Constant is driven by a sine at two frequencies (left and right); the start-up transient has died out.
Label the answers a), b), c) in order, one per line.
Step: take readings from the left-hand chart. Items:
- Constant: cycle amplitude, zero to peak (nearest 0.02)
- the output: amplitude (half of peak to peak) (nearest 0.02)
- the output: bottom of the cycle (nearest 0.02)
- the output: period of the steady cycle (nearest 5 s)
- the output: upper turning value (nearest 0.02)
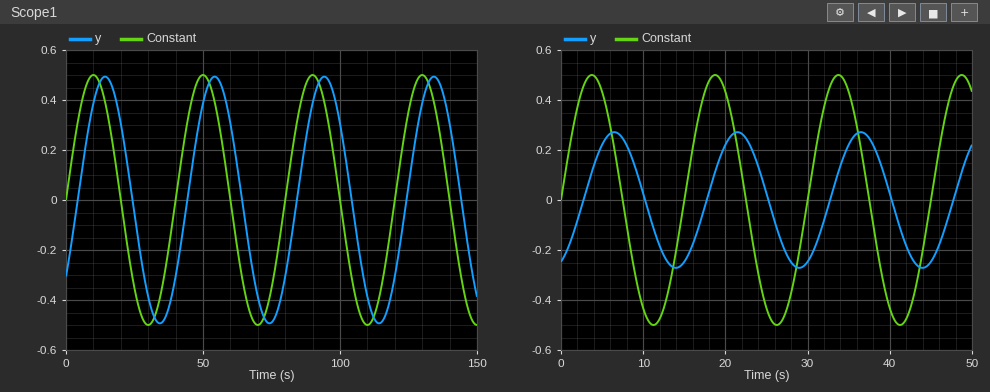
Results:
a) 0.50
b) 0.50
c) -0.50
d) 40 s
e) 0.50
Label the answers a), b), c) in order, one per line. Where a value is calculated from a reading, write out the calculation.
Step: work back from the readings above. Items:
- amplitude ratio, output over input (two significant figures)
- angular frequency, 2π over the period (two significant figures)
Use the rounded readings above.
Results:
a) 0.5 / 0.5 = 1.0
b) 2π / 40 = 0.16 rad/s
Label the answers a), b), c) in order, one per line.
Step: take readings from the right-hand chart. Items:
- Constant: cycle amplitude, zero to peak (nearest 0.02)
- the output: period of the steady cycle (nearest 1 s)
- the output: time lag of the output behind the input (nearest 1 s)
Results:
a) 0.50
b) 15 s
c) 3 s
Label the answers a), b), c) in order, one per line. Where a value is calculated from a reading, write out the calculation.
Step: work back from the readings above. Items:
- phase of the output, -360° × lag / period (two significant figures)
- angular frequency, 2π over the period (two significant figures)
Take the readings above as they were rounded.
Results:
a) -360 × 3 / 15 = -72°
b) 2π / 15 = 0.42 rad/s
